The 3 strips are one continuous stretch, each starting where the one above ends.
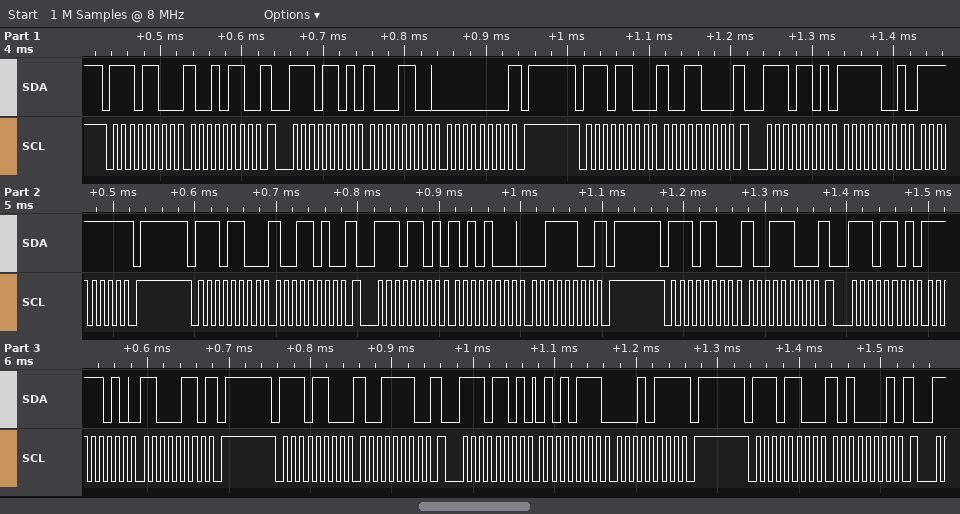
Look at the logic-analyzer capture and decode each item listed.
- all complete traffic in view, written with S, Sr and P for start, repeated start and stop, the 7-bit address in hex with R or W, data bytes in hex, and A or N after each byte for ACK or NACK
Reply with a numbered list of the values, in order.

1. S 76W A 96 A Sr 76R A 8C A 00 N P S 76W A 98 A Sr 76R A F9 A FF N P S 76W A 9A A Sr 76R A A8 A 3C N P S 76W A 9C A Sr 76R A FA A C6 N P S 76W A 9E A Sr 76R A 57 A 17 N P S 76W A A1 A
